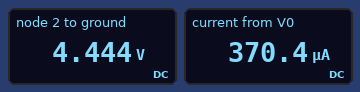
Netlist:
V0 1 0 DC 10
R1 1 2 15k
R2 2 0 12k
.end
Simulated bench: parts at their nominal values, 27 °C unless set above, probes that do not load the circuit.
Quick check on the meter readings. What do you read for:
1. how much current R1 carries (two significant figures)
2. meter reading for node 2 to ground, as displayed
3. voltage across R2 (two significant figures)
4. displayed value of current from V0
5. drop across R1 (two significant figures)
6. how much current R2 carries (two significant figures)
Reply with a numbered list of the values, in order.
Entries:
1. 370 µA
2. 4.444 V
3. 4.4 V
4. 370.4 µA
5. 5.6 V
6. 370 µA
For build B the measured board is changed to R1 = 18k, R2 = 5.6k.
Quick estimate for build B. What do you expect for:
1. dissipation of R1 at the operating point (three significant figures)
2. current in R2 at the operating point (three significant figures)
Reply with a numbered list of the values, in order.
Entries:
1. 3.23 mW
2. 424 µA
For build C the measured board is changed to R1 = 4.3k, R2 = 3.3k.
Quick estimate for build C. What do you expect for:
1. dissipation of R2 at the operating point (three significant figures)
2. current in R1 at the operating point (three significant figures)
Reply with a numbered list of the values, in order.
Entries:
1. 5.71 mW
2. 1.32 mA
